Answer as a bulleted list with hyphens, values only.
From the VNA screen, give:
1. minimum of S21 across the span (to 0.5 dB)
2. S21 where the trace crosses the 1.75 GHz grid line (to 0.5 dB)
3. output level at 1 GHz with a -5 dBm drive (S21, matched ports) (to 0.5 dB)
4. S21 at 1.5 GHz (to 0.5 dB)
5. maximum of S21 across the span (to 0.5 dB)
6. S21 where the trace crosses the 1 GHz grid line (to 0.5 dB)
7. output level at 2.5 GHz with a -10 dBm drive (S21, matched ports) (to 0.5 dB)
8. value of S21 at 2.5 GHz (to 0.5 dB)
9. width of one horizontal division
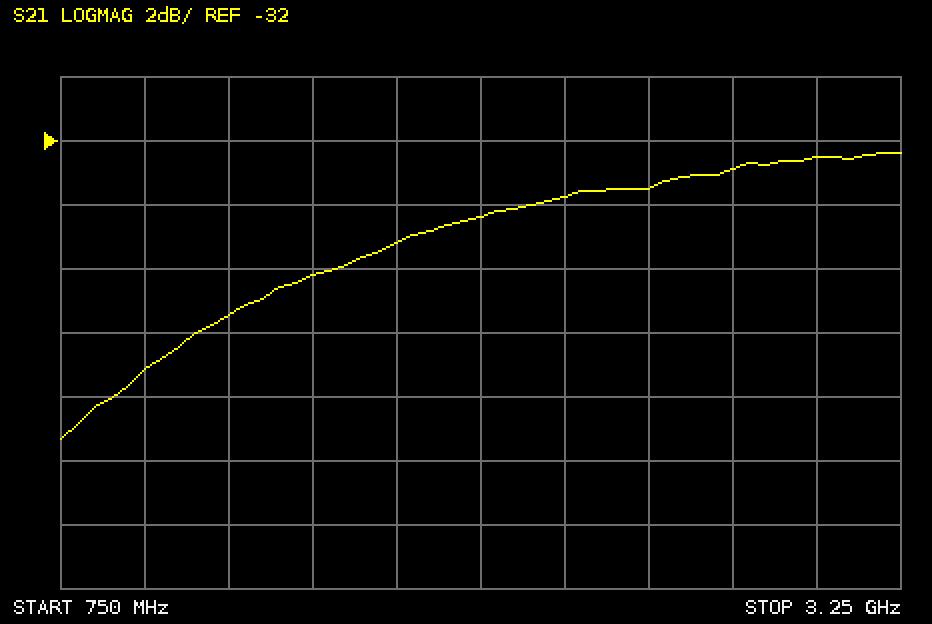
- -41.5 dB
- -35.0 dB
- -44.0 dBm
- -36.0 dB
- -32.5 dB
- -39.0 dB
- -43.5 dBm
- -33.5 dB
- 250 MHz
